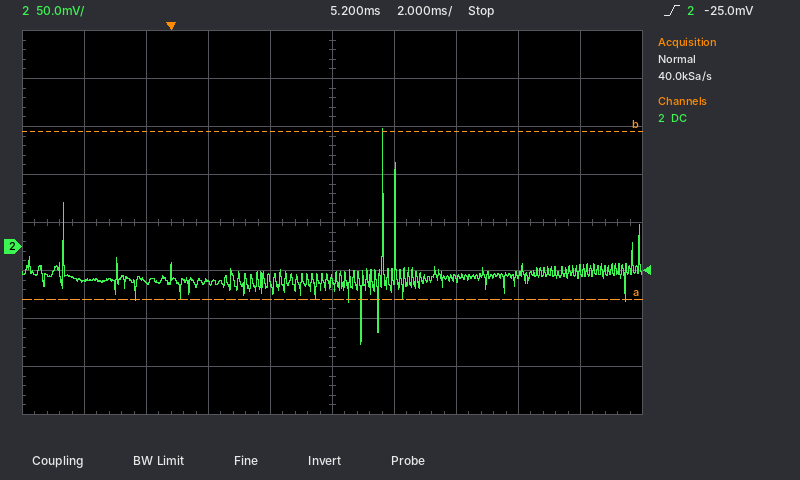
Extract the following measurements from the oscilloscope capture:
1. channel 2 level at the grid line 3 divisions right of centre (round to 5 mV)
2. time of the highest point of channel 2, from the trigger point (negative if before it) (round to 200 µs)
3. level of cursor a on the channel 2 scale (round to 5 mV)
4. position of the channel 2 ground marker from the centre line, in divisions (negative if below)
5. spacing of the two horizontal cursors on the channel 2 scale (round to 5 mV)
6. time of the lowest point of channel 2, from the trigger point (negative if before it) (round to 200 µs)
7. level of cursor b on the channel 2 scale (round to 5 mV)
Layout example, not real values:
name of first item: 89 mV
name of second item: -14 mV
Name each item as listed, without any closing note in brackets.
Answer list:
channel 2 level at the grid line 3 divisions right of centre: -30 mV
time of the highest point of channel 2, from the trigger point (negative if before it): +6.8 ms
level of cursor a on the channel 2 scale: -55 mV
position of the channel 2 ground marker from the centre line, in divisions: -0.5 div
spacing of the two horizontal cursors on the channel 2 scale: 175 mV
time of the lowest point of channel 2, from the trigger point (negative if before it): +6.2 ms
level of cursor b on the channel 2 scale: 120 mV
